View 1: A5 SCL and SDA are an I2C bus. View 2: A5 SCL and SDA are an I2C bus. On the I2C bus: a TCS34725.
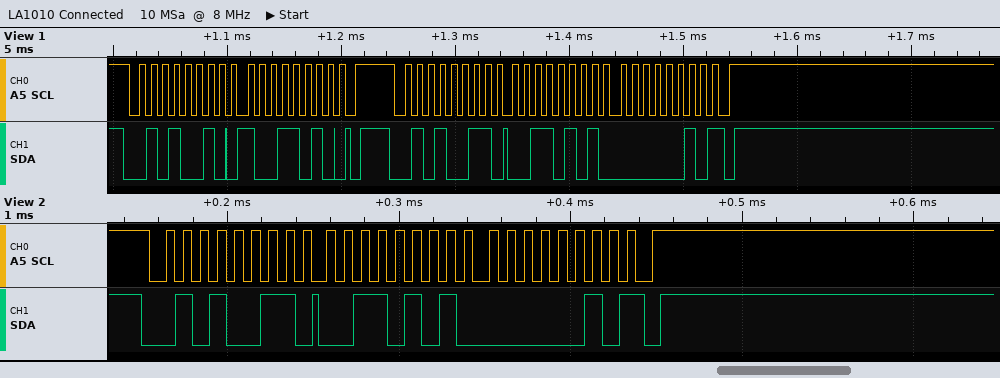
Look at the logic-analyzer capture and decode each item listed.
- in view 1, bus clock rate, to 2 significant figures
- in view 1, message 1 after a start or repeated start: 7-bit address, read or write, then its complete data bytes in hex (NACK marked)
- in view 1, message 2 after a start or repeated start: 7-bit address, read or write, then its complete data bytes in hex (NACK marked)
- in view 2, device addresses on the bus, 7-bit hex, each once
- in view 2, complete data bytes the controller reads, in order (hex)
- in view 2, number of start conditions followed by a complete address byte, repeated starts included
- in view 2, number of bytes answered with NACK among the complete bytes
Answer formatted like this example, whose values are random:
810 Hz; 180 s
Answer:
100 kHz; 0x29 write: 9A; 0x29 read: 35 02 NACK; 0x29; 35 02; 1; 1
